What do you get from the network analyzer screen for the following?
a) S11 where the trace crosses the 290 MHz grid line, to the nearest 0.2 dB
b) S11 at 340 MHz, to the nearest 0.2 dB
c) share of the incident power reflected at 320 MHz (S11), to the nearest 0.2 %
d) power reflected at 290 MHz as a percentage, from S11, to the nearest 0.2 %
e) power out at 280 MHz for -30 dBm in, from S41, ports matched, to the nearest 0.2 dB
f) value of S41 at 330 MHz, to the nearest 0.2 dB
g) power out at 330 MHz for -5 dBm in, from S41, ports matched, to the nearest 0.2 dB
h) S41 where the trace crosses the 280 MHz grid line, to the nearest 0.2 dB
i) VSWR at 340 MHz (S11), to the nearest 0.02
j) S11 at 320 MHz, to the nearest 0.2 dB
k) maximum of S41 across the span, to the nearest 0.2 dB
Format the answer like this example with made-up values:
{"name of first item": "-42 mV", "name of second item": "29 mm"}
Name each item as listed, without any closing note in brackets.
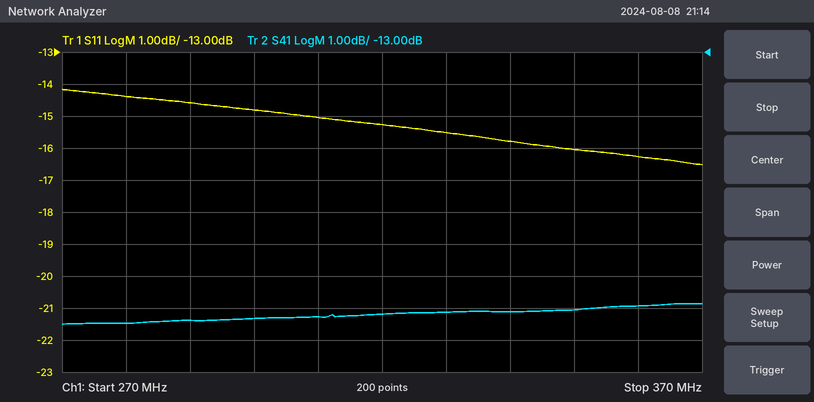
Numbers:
{"S11 where the trace crosses the 290 MHz grid line, to the nearest 0.2 dB": "-14.6 dB", "S11 at 340 MHz, to the nearest 0.2 dB": "-15.8 dB", "share of the incident power reflected at 320 MHz (S11), to the nearest 0.2 %": "3.0 %", "power reflected at 290 MHz as a percentage, from S11, to the nearest 0.2 %": "3.4 %", "power out at 280 MHz for -30 dBm in, from S41, ports matched, to the nearest 0.2 dB": "-51.4 dBm", "value of S41 at 330 MHz, to the nearest 0.2 dB": "-21.2 dB", "power out at 330 MHz for -5 dBm in, from S41, ports matched, to the nearest 0.2 dB": "-26.2 dBm", "S41 where the trace crosses the 280 MHz grid line, to the nearest 0.2 dB": "-21.4 dB", "VSWR at 340 MHz (S11), to the nearest 0.02": "1.38", "S11 at 320 MHz, to the nearest 0.2 dB": "-15.2 dB", "maximum of S41 across the span, to the nearest 0.2 dB": "-20.8 dB"}
